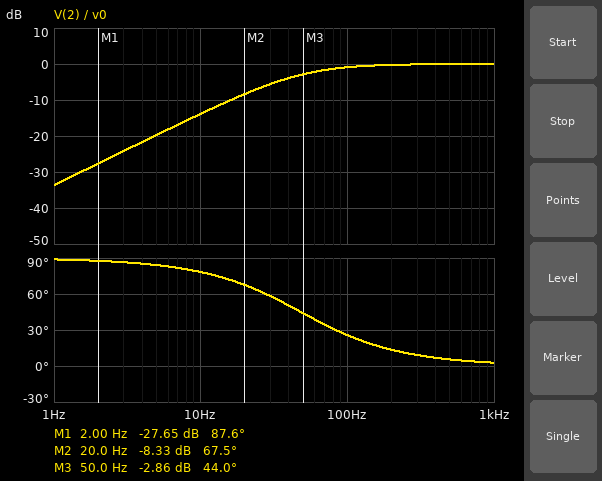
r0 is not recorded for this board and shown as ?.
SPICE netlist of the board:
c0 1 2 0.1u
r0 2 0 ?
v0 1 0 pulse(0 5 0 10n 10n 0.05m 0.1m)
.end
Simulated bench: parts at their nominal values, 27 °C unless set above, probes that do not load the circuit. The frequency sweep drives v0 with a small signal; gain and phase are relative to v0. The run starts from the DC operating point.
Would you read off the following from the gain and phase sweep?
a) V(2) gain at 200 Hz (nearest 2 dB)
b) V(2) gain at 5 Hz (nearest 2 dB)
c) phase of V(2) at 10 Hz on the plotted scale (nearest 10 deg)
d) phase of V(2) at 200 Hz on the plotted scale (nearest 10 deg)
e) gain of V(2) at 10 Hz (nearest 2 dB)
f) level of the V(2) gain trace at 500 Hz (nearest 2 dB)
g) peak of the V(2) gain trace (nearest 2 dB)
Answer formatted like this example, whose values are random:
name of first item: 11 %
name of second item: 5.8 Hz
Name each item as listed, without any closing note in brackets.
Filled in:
V(2) gain at 200 Hz: 0 dB
V(2) gain at 5 Hz: -20 dB
phase of V(2) at 10 Hz on the plotted scale: 80 deg
phase of V(2) at 200 Hz on the plotted scale: 10 deg
gain of V(2) at 10 Hz: -14 dB
level of the V(2) gain trace at 500 Hz: 0 dB
peak of the V(2) gain trace: 0 dB
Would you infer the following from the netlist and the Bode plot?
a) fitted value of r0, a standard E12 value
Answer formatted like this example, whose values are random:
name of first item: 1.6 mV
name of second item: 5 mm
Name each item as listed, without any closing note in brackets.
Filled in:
fitted value of r0, a standard E12 value: 33 kΩ
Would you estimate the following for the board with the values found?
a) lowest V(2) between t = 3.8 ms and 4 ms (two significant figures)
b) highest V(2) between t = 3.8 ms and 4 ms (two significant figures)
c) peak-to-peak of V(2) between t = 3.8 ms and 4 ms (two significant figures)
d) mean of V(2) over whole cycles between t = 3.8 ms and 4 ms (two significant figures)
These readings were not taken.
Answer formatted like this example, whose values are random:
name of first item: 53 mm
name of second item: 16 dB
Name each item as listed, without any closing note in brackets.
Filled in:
lowest V(2) between t = 3.8 ms and 4 ms: -1.8 V
highest V(2) between t = 3.8 ms and 4 ms: 3.3 V
peak-to-peak of V(2) between t = 3.8 ms and 4 ms: 5.1 V
mean of V(2) over whole cycles between t = 3.8 ms and 4 ms: 760 mV
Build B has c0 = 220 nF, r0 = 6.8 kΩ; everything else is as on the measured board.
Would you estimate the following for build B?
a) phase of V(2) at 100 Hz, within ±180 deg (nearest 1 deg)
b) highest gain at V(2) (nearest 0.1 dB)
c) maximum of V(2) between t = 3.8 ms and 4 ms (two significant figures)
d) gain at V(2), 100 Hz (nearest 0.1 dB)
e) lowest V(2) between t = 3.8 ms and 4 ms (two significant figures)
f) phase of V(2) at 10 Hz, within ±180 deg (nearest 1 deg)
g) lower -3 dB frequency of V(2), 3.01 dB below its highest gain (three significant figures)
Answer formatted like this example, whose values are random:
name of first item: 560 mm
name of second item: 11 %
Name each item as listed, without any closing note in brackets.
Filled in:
phase of V(2) at 100 Hz, within ±180 deg: 47 deg
highest gain at V(2): 0 dB
maximum of V(2) between t = 3.8 ms and 4 ms: 2.7 V
gain at V(2), 100 Hz: -3.3 dB
lowest V(2) between t = 3.8 ms and 4 ms: -2.4 V
phase of V(2) at 10 Hz, within ±180 deg: 85 deg
lower -3 dB frequency of V(2), 3.01 dB below its highest gain: 106 Hz
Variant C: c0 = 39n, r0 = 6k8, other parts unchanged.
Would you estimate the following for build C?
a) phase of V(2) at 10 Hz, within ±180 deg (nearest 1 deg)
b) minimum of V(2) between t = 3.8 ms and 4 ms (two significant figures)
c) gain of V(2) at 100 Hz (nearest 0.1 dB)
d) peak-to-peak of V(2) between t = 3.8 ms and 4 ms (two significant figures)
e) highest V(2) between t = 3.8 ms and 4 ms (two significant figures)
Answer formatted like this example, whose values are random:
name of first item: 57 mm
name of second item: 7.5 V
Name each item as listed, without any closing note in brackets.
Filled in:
phase of V(2) at 10 Hz, within ±180 deg: 89 deg
minimum of V(2) between t = 3.8 ms and 4 ms: -2.7 V
gain of V(2) at 100 Hz: -15.7 dB
peak-to-peak of V(2) between t = 3.8 ms and 4 ms: 5.5 V
highest V(2) between t = 3.8 ms and 4 ms: 2.7 V
